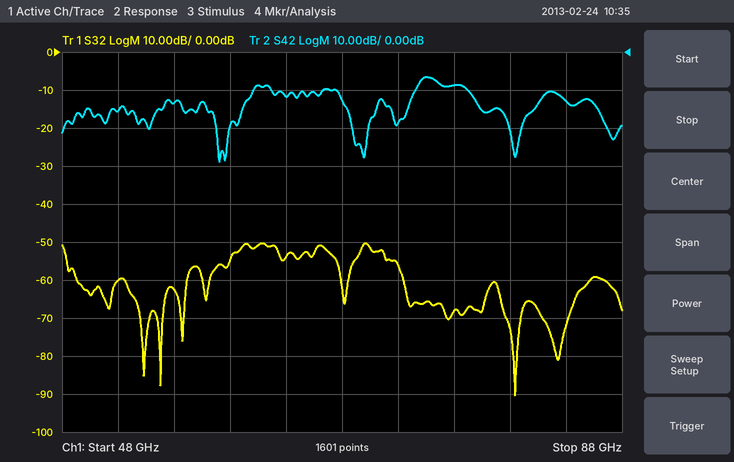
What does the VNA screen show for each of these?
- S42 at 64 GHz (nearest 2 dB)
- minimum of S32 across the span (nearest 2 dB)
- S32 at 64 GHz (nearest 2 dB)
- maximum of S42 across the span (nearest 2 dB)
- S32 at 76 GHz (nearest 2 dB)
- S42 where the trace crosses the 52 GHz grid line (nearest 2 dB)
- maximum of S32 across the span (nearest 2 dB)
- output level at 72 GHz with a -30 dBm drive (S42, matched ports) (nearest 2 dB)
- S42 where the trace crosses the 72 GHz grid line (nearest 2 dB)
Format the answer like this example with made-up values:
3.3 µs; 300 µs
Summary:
-12 dB; -90 dB; -54 dB; -6 dB; -68 dB; -16 dB; -50 dB; -48 dBm; -18 dB
